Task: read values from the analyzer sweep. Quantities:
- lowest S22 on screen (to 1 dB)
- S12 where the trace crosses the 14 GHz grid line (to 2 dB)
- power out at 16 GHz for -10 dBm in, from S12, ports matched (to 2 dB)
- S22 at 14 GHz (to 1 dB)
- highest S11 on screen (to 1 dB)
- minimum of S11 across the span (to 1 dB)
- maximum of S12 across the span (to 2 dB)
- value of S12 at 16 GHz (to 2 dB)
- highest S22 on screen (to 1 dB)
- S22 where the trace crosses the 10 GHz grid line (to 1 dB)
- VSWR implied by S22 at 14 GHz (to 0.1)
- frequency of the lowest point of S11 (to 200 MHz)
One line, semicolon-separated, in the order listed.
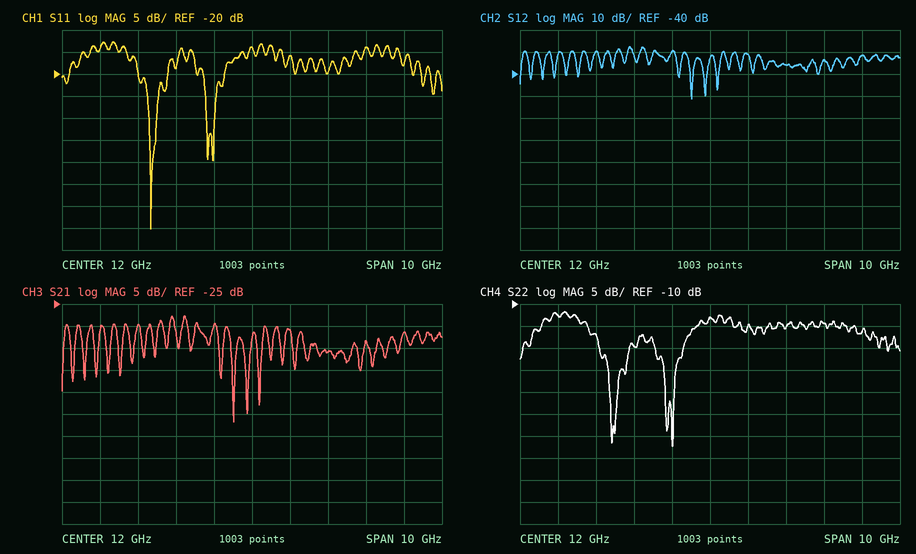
-42 dB; -36 dB; -42 dBm; -15 dB; -13 dB; -55 dB; -28 dB; -32 dB; -12 dB; -20 dB; 1.4; 9.4 GHz
